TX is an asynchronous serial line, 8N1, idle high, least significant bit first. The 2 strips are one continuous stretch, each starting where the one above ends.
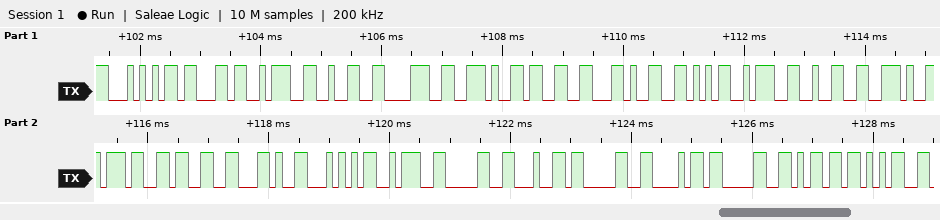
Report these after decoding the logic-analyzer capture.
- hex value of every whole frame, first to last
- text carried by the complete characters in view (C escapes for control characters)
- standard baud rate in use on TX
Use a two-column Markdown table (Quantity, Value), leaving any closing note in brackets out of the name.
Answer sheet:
| Quantity | Value |
|---|---|
| hex value of every whole frame, first to last | 54 63 3A 32 38 2E 33 2C 56 3A 32 2E 37 33 2C 54 3A 30 64 30 68 30 6D 35 |
| text carried by the complete characters in view | "Tc:28.3,V:2.73,T:0d0h0m5" |
| standard baud rate in use on TX | 9600 baud |
